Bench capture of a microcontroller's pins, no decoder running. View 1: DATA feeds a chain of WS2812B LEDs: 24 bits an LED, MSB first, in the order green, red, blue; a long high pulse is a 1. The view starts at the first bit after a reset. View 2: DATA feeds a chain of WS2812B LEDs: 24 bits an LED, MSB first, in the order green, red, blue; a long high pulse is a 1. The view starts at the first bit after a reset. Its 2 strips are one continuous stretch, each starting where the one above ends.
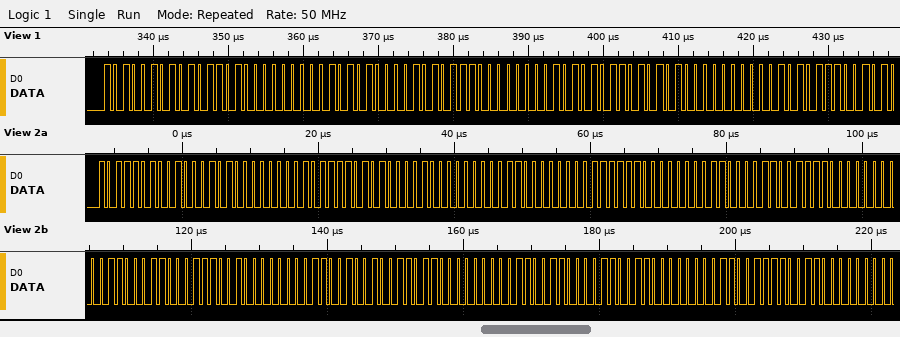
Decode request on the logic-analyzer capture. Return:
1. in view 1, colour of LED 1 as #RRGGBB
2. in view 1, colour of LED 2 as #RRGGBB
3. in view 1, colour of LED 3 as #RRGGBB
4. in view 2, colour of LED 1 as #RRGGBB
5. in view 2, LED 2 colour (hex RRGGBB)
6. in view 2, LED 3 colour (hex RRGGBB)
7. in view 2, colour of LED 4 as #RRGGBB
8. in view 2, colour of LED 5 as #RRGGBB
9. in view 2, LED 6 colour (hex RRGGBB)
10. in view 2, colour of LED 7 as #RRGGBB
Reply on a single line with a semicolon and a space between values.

#5AA500; #57A800; #54AB00; #45BA00; #42BD00; #3FC000; #3CC300; #39C600; #36C900; #33CC00
